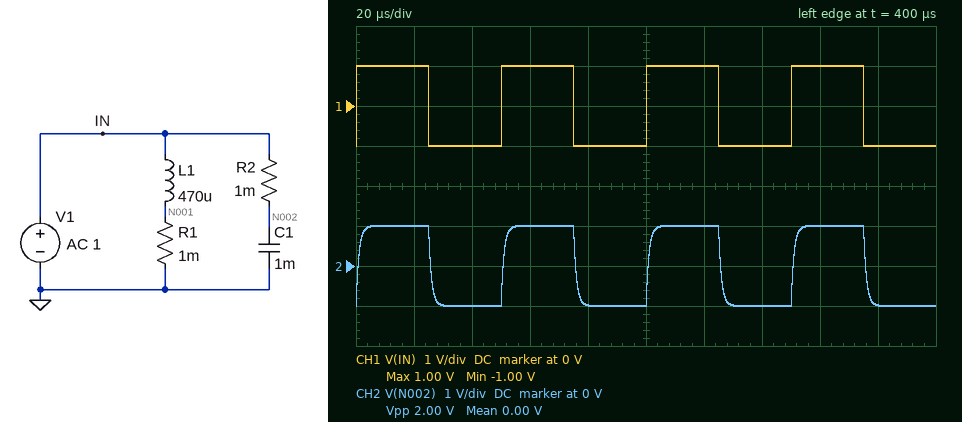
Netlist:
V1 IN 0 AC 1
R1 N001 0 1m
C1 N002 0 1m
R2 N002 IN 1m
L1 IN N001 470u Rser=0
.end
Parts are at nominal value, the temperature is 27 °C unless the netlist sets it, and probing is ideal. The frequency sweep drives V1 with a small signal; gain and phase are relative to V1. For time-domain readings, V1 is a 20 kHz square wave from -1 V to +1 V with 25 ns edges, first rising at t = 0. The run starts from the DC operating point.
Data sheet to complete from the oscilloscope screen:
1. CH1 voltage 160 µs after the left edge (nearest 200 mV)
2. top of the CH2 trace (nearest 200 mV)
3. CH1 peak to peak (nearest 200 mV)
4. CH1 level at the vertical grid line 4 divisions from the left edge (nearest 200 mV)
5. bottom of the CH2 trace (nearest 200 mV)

1.0 V
1.0 V
2.0 V
-1.0 V
-1.0 V
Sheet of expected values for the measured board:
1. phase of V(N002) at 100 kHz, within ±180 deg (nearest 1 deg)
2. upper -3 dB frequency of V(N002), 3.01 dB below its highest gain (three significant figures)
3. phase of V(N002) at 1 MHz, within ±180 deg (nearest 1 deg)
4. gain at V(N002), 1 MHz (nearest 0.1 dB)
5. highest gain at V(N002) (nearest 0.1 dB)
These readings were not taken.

-32 deg
159 kHz
-81 deg
-16.1 dB
0 dB
